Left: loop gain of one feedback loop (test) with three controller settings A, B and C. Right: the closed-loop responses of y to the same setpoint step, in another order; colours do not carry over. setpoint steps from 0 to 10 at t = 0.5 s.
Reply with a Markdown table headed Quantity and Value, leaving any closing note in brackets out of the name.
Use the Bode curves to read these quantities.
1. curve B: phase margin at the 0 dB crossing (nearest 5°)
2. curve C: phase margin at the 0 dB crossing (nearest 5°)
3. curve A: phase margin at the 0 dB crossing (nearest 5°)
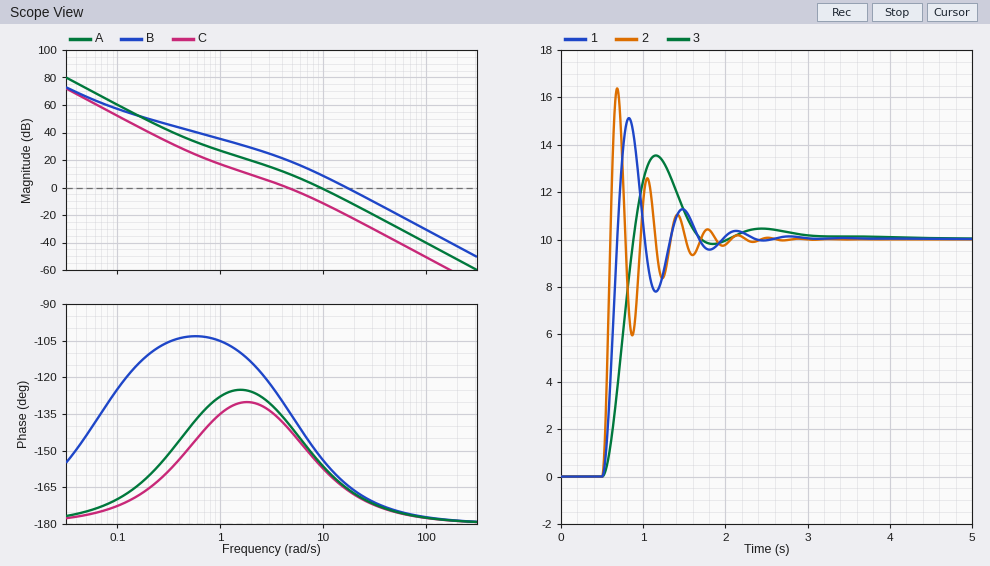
| Quantity | Value |
|---|---|
| curve B: phase margin at the 0 dB crossing | 15° |
| curve C: phase margin at the 0 dB crossing | 40° |
| curve A: phase margin at the 0 dB crossing | 25° |
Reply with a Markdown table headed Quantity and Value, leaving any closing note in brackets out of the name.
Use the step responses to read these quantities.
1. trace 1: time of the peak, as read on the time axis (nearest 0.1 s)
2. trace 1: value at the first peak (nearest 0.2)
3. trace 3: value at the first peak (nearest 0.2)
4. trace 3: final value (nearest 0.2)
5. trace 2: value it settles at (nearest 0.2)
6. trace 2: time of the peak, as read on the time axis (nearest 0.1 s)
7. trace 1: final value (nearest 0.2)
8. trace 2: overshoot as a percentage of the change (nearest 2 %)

| Quantity | Value |
|---|---|
| trace 1: time of the peak, as read on the time axis | 0.8 s |
| trace 1: value at the first peak | 15.2 |
| trace 3: value at the first peak | 13.6 |
| trace 3: final value | 10.0 |
| trace 2: value it settles at | 10.0 |
| trace 2: time of the peak, as read on the time axis | 0.7 s |
| trace 1: final value | 10.0 |
| trace 2: overshoot as a percentage of the change | 64 % |
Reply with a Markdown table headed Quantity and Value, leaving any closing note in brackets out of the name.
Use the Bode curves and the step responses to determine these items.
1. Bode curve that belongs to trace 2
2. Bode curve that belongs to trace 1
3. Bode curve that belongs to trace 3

| Quantity | Value |
|---|---|
| Bode curve that belongs to trace 2 | B |
| Bode curve that belongs to trace 1 | A |
| Bode curve that belongs to trace 3 | C |
